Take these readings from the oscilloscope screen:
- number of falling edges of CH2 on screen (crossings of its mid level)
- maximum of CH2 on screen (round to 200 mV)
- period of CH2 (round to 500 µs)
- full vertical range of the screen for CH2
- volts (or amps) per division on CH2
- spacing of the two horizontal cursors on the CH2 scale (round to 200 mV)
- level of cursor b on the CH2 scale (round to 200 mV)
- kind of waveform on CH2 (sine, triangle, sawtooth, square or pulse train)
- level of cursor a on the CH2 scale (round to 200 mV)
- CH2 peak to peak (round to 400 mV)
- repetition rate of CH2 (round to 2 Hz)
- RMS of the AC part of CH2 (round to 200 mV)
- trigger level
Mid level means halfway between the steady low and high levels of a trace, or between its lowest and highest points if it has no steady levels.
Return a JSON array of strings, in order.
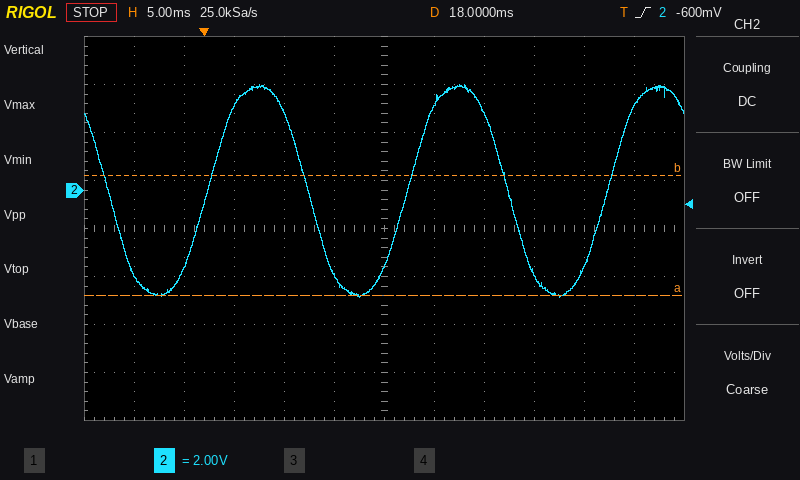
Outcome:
["3", "4.4 V", "20.0 ms", "16 V", "2 V", "5.0 V", "600 mV", "sine", "-4.4 V", "8.8 V", "50 Hz", "3.2 V", "-600 mV"]
